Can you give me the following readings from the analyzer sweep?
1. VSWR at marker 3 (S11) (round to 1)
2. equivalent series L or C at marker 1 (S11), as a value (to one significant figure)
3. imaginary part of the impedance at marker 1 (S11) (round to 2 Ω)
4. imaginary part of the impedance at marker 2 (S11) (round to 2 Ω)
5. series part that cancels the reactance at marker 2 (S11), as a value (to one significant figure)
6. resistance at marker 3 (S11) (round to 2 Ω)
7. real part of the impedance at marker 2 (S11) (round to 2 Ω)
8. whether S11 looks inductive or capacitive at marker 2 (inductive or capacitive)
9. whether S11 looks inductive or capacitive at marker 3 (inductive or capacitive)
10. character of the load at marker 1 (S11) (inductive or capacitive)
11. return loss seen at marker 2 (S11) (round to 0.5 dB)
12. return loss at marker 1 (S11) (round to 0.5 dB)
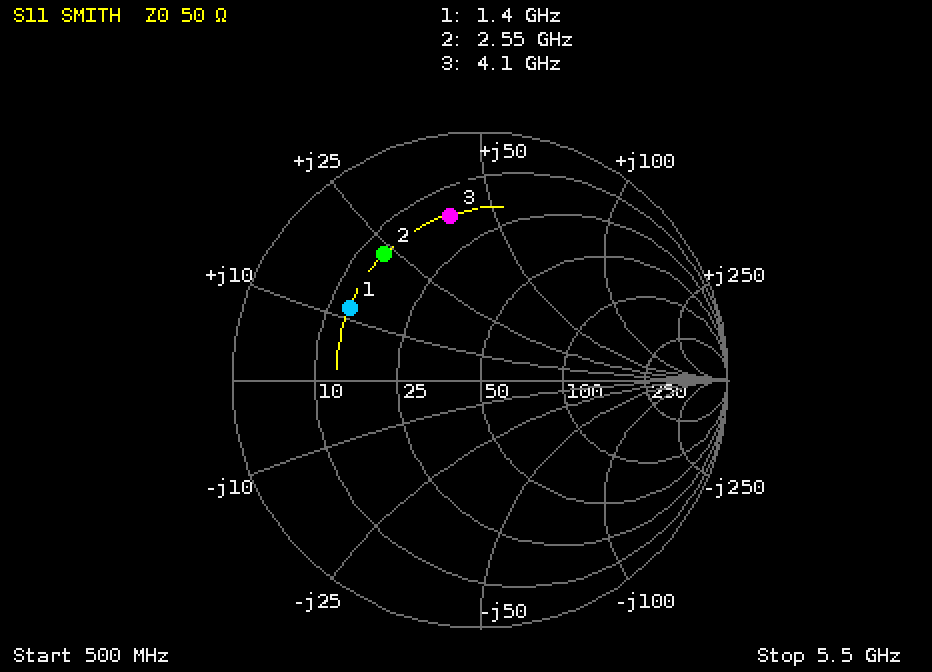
5
1 nH
+12 Ω
+24 Ω
3 pF
16 Ω
14 Ω
inductive
inductive
inductive
4.0 dB
4.5 dB
